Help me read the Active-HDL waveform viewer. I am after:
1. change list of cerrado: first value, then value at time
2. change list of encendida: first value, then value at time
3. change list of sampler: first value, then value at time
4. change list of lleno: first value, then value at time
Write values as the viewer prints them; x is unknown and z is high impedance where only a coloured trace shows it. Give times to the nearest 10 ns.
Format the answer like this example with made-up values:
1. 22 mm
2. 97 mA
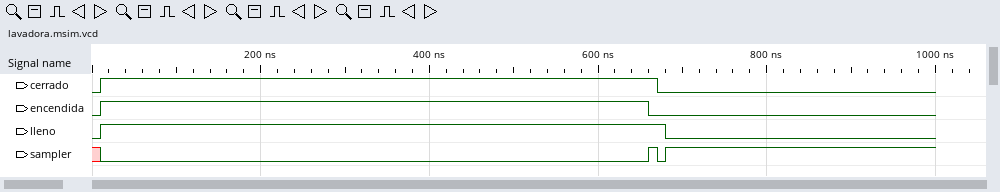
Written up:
1. 0, 1 at 10 ns, 0 at 670 ns
2. 0, 1 at 10 ns, 0 at 660 ns
3. x, 0 at 10 ns, 1 at 660 ns, 0 at 670 ns, 1 at 680 ns
4. 0, 1 at 10 ns, 0 at 680 ns
